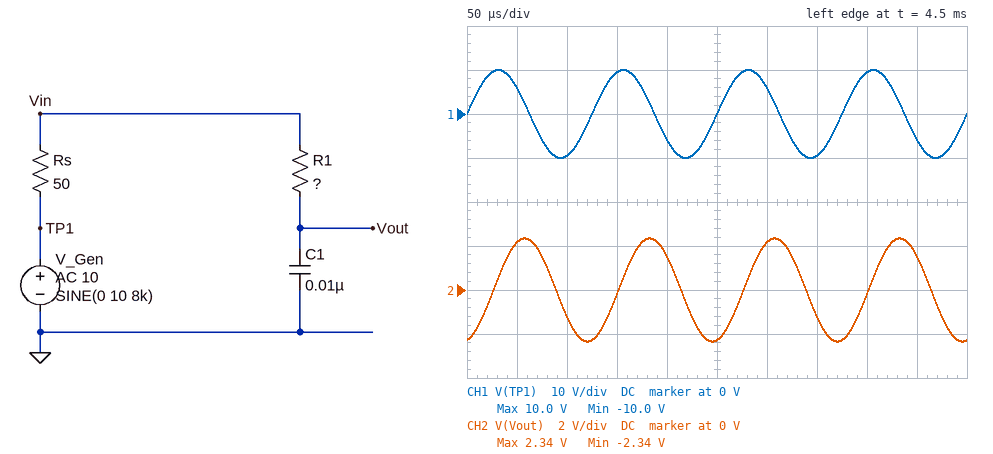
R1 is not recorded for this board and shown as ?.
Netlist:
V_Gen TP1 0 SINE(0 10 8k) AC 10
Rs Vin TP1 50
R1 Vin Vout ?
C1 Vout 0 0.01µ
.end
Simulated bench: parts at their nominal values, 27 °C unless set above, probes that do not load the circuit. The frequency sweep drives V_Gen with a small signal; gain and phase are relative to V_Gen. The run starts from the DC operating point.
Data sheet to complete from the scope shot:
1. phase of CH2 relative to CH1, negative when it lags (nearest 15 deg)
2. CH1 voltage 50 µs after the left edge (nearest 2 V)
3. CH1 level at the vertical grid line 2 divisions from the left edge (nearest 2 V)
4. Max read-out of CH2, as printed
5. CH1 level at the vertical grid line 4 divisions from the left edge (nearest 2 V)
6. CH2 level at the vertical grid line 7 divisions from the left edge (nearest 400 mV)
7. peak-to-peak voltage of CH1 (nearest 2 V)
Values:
-75 deg
6 V
-10 V
2.34 V
-6 V
-1.2 V
20 V
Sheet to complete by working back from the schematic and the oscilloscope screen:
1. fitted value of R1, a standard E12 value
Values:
8.2 kΩ
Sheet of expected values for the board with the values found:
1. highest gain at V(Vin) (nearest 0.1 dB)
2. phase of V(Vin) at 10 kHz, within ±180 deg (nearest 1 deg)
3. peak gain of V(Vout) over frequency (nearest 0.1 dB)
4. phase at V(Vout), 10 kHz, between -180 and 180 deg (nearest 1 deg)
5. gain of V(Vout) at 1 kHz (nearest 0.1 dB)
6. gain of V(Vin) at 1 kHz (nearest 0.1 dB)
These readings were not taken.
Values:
0 dB
0 deg
0 dB
-79 deg
-1.0 dB
0 dB
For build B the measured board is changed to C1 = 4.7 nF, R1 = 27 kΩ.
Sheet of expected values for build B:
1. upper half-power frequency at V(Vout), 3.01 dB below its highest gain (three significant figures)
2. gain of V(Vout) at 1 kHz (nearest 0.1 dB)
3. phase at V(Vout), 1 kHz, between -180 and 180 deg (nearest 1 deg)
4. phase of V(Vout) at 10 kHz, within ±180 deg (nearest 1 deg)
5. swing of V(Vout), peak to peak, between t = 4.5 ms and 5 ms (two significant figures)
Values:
1.25 kHz
-2.1 dB
-39 deg
-83 deg
3.1 V
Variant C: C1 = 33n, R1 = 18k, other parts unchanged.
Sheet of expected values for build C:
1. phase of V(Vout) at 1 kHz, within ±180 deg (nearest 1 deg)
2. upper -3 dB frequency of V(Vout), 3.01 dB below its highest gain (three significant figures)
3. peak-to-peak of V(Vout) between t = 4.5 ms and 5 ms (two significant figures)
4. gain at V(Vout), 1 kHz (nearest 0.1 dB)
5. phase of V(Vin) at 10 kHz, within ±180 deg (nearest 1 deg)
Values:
-75 deg
267 Hz
670 mV
-11.8 dB
0 deg
